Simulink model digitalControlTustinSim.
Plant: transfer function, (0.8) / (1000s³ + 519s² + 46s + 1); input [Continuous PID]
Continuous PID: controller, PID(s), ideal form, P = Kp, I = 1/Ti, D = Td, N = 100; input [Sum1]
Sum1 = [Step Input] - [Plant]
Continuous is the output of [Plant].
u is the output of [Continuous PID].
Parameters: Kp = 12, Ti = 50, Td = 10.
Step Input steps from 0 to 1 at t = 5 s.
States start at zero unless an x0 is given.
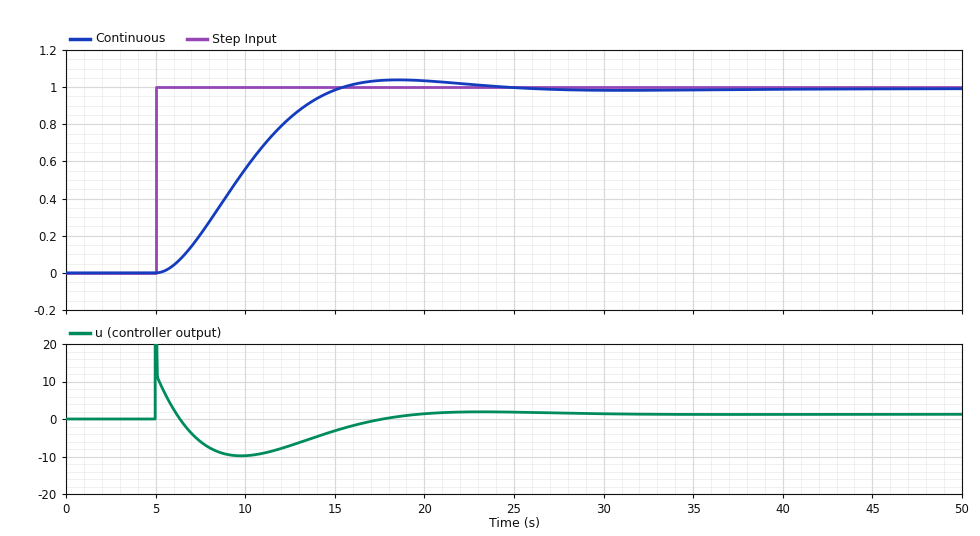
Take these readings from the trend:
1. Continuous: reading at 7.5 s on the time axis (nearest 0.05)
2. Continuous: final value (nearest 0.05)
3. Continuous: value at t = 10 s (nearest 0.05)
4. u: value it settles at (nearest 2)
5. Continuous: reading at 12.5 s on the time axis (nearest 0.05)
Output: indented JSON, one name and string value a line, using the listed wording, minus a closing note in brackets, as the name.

{
  "Continuous: reading at 7.5 s on the time axis": "0.20",
  "Continuous: final value": "1.00",
  "Continuous: value at t = 10 s": "0.55",
  "u: value it settles at": "2",
  "Continuous: reading at 12.5 s on the time axis": "0.85"
}
